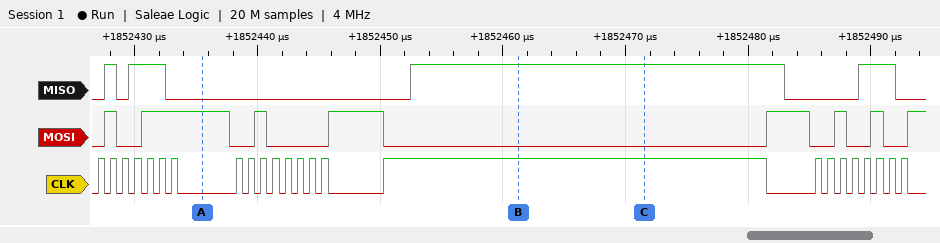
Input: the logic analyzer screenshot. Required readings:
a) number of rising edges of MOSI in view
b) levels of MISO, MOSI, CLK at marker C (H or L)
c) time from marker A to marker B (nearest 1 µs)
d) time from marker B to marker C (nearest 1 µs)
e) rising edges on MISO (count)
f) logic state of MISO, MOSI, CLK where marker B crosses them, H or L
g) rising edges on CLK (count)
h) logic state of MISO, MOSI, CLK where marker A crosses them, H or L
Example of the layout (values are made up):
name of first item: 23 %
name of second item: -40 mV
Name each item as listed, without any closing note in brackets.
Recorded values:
number of rising edges of MOSI in view: 8
levels of MISO, MOSI, CLK at marker C: MISO=H, MOSI=L, CLK=H
time from marker A to marker B: 26 µs
time from marker B to marker C: 10 µs
rising edges on MISO: 4
logic state of MISO, MOSI, CLK where marker B crosses them, H or L: MISO=H, MOSI=L, CLK=H
rising edges on CLK: 24
logic state of MISO, MOSI, CLK where marker A crosses them, H or L: MISO=L, MOSI=H, CLK=L
